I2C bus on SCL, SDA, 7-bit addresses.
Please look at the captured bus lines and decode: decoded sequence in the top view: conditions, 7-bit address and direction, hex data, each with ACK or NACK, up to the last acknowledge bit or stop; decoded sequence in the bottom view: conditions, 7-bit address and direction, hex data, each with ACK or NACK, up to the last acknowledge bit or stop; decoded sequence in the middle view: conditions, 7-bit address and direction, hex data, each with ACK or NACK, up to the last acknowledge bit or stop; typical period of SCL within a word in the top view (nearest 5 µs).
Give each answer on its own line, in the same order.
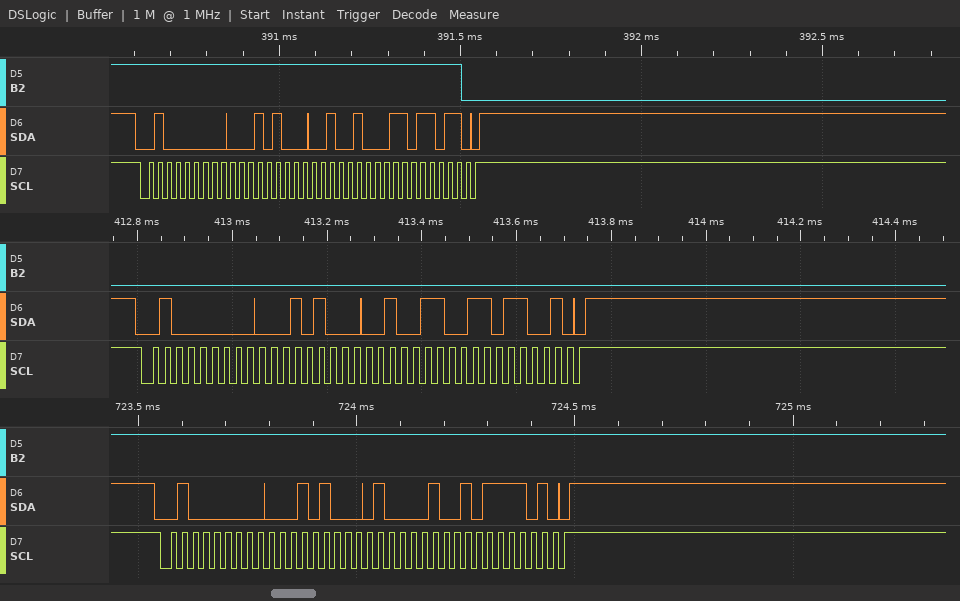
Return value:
start, address 20 write ACK, 14 ACK, 24 ACK, DB ACK, stop
start, address 20 write ACK, 14 ACK, 42 ACK, BD ACK, stop
start, address 20 write ACK, 14 ACK, 26 ACK, D9 ACK, stop
25 µs
